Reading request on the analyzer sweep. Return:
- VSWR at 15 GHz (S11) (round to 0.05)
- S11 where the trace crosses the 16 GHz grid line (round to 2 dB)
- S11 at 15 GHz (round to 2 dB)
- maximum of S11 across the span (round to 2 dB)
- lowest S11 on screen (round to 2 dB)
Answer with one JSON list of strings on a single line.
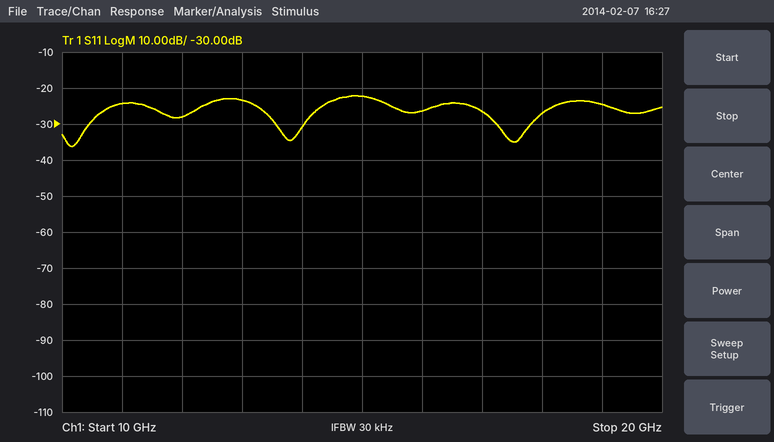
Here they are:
["1.15", "-26 dB", "-22 dB", "-22 dB", "-36 dB"]
